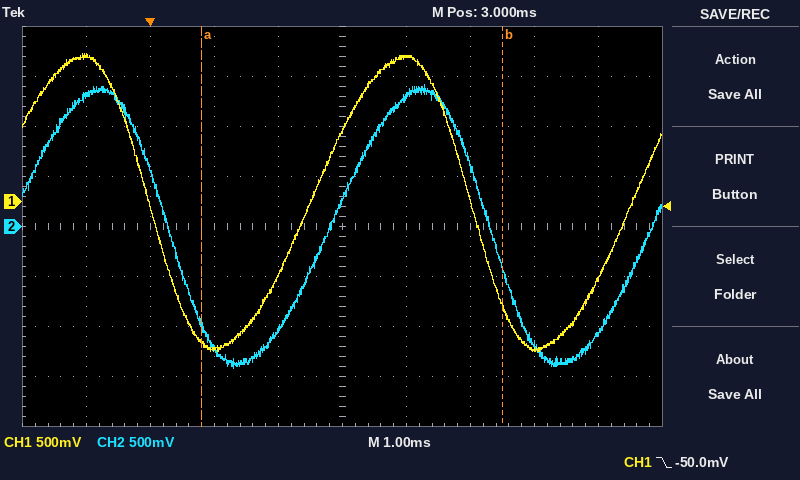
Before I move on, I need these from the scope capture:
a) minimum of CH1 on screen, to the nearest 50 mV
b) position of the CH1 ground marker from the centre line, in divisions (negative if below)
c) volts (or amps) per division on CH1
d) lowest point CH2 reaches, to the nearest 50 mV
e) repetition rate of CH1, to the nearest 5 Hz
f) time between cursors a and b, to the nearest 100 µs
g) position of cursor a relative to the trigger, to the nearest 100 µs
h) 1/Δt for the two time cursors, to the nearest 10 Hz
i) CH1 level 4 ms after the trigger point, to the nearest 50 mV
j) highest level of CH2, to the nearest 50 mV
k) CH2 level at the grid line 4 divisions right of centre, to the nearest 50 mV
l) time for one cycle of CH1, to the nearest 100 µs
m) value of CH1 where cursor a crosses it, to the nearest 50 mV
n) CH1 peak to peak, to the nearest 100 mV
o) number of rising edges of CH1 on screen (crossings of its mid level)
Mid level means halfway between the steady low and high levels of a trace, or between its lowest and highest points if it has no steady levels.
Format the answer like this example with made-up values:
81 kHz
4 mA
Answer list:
-1.50 V
+0.5 div
500 mV
-1.40 V
200 Hz
4.7 ms
+800 µs
210 Hz
1.45 V
1.40 V
-1.05 V
5.0 ms
-1.40 V
3.00 V
2
